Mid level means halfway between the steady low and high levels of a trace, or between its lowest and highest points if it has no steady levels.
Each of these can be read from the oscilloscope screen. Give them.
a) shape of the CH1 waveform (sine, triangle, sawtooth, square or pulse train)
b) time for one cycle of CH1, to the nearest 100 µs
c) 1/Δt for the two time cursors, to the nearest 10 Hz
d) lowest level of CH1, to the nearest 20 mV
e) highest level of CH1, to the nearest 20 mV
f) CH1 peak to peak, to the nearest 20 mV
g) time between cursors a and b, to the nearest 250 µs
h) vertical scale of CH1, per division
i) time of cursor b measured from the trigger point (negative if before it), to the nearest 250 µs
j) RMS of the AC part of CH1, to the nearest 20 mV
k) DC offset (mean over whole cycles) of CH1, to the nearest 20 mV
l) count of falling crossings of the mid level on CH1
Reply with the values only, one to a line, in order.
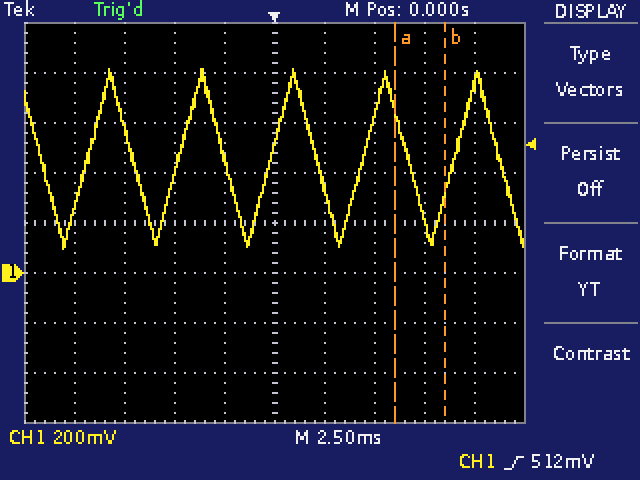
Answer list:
triangle
4.6 ms
400 Hz
100 mV
820 mV
720 mV
2.50 ms
200 mV
+8.50 ms
200 mV
460 mV
6
